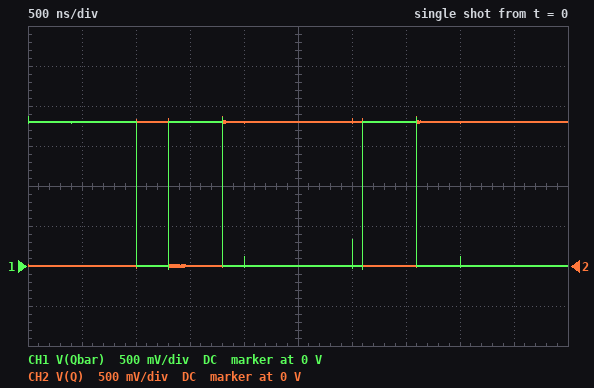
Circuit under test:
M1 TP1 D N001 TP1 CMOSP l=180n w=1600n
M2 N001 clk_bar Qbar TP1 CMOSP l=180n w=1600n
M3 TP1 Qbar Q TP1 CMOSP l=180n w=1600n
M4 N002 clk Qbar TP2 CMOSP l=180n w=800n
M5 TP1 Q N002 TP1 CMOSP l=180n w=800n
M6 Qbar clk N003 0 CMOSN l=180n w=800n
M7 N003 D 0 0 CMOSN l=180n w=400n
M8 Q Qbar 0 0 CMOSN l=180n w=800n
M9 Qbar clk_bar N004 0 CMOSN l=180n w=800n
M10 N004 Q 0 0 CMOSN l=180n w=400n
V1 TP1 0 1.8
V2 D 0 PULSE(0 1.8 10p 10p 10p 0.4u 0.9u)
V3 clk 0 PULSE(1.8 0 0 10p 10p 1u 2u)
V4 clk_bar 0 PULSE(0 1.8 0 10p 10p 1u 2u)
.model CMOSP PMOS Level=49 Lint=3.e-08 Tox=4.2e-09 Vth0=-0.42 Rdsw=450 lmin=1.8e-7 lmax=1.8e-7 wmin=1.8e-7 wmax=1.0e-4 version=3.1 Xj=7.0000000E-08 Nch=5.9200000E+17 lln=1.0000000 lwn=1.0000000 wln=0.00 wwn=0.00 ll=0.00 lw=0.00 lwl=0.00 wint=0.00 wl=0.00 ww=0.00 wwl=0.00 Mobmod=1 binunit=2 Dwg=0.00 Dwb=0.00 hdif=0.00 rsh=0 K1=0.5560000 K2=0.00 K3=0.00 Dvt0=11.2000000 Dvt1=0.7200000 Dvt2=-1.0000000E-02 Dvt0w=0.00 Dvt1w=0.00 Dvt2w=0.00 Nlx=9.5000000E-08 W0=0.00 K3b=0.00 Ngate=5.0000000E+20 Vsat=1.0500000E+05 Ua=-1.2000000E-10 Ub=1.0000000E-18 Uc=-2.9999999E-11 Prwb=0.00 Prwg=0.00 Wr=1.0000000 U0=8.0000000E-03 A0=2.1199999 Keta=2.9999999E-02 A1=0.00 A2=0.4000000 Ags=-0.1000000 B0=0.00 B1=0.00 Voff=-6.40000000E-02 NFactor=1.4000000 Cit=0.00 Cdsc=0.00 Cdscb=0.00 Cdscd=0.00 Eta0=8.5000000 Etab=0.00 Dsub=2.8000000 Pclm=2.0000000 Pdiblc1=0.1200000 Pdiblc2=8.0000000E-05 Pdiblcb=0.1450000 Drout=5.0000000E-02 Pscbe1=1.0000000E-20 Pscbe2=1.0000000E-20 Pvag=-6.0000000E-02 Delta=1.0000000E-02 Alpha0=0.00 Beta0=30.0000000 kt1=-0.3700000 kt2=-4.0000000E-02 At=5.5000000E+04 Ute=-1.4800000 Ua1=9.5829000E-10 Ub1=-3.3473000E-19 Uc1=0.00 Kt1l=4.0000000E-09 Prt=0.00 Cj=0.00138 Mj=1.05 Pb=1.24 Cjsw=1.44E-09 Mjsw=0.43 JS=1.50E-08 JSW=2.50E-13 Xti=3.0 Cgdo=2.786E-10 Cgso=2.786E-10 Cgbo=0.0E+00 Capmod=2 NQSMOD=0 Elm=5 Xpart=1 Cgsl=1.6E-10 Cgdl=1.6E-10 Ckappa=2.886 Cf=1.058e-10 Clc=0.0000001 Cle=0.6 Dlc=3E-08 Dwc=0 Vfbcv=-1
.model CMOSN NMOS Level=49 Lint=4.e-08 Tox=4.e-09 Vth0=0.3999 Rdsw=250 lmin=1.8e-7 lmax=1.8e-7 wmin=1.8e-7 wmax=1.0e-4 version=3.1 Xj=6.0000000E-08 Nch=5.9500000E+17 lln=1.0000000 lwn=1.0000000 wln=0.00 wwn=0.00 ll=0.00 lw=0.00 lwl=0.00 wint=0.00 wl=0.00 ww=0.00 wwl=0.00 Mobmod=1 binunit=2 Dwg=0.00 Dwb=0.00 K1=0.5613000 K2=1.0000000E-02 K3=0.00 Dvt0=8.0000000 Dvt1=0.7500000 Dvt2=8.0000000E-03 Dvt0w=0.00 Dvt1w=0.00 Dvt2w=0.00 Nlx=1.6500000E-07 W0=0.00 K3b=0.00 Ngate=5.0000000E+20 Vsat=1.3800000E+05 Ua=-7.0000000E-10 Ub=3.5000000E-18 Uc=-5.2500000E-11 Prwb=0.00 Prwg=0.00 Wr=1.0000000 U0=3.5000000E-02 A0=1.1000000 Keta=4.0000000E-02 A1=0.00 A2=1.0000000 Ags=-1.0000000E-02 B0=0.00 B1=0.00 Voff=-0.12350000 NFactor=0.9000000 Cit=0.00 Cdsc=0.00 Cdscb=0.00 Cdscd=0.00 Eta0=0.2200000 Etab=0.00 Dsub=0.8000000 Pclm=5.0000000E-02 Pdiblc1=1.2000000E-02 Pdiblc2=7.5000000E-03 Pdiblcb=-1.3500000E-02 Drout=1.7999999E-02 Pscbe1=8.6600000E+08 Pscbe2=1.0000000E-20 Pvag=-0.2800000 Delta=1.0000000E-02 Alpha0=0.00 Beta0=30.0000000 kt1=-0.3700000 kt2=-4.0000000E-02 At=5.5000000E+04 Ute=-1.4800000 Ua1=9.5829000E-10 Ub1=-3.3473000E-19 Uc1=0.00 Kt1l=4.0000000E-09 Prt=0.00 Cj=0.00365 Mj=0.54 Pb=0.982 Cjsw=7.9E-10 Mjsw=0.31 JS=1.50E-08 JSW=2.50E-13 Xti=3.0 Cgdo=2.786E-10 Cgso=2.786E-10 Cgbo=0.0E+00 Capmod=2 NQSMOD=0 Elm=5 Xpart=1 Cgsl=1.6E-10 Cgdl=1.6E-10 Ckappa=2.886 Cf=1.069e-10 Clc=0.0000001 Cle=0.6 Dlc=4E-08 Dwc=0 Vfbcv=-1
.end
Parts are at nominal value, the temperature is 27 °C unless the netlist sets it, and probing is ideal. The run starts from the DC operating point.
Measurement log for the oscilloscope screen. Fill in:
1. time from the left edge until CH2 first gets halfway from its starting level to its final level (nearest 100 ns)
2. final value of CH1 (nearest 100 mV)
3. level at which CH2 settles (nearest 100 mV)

1.0 µs
0 V
1.8 V
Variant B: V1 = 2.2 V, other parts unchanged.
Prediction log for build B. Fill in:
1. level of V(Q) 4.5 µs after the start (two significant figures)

2.2 V
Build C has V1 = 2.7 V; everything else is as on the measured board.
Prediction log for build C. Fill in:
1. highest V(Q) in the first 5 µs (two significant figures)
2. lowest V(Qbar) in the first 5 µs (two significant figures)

2.7 V
170 mV
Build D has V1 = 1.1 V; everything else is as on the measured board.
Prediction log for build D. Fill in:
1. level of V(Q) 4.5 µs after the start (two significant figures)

1.1 V
